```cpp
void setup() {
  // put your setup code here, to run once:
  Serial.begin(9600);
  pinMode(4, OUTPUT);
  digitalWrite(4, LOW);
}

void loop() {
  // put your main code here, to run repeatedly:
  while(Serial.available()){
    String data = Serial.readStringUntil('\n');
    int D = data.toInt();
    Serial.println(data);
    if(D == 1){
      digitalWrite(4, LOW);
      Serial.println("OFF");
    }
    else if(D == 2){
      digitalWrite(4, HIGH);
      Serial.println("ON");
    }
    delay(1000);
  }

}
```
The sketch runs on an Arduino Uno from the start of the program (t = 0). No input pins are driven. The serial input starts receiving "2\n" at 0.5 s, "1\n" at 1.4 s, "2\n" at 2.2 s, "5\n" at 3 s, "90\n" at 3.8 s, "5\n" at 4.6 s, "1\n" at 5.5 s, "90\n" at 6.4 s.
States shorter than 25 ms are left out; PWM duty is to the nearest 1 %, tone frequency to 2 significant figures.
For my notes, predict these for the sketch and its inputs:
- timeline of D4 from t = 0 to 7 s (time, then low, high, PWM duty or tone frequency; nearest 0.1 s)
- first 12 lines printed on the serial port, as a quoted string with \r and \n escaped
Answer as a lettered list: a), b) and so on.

a) 0 s low; 0.5 s high; 1.5 s low; 2.5 s high; 6.5 s low
b) "2\r\nON\r\n1\r\nOFF\r\n2\r\nON\r\n5\r\n90\r\n5\r\n1\r\nOFF\r\n90\r\n"
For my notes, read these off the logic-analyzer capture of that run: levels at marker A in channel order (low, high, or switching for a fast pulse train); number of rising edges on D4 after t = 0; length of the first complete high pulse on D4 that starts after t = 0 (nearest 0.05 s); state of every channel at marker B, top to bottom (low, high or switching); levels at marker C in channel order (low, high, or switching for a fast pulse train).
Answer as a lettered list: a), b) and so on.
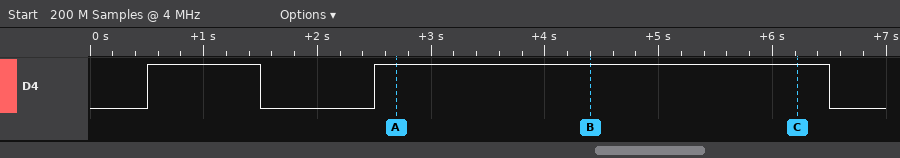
a) D4 high
b) 2
c) 1.00 s
d) D4 high
e) D4 high
